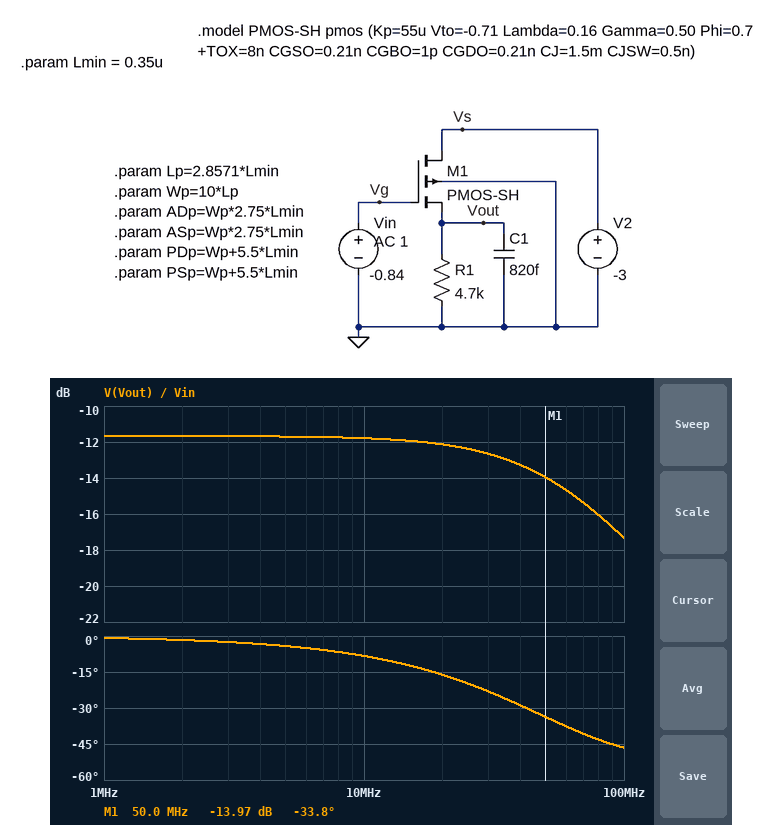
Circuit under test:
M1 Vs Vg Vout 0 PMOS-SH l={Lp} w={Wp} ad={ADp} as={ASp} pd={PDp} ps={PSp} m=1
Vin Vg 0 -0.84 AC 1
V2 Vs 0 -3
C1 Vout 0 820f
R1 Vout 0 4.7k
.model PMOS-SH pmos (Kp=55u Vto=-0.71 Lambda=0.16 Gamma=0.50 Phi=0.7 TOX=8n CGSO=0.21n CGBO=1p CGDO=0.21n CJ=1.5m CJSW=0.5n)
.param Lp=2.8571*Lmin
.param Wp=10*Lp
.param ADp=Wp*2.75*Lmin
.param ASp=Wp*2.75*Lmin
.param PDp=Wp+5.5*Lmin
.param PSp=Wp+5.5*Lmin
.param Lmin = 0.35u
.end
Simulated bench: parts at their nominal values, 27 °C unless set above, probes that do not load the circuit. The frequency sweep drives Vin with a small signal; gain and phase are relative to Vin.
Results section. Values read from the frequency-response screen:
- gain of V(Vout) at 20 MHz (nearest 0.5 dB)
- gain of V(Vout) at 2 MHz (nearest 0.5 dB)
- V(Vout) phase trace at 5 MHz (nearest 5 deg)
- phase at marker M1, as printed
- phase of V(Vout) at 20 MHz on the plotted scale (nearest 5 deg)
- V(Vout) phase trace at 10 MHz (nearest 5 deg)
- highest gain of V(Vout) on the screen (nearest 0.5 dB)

-12.0 dB
-11.5 dB
-5 deg
-33.8 deg
-15 deg
-10 deg
-11.5 dB
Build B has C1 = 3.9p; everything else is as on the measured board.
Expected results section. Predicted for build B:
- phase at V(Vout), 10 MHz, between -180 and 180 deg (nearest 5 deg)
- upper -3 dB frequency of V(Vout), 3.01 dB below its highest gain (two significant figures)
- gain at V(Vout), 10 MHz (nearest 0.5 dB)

-35 deg
13 MHz
-13.5 dB
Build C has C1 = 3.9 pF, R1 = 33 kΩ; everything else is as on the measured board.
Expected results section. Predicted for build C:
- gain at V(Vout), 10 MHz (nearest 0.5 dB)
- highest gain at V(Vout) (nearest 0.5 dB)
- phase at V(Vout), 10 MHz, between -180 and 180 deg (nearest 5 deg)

-14.5 dB
-5.5 dB
-65 deg
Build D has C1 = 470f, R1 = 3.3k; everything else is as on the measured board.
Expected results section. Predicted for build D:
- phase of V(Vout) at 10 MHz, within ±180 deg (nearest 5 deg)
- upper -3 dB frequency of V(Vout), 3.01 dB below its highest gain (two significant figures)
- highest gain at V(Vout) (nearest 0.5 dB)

-5 deg
140 MHz
-13.5 dB
